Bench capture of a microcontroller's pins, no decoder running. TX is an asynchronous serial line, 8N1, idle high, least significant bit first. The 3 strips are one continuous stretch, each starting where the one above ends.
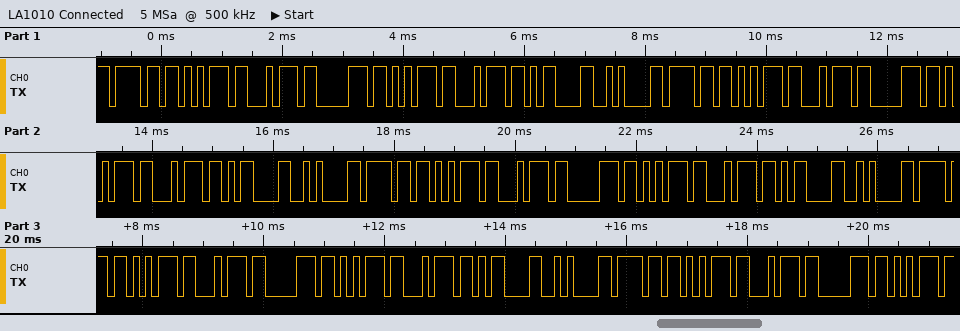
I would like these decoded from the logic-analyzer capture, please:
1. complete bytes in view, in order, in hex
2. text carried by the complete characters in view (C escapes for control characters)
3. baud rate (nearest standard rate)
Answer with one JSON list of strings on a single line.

["6F 75 74 70 75 74 0D 0A 6F 75 74 70 75 74 0D 0A 6F 75 74 70 75 74 0D 0A 6F 75 74 70 75 74 0D 0A 6F 75 74 70 75", "\"output\\r\\noutput\\r\\noutput\\r\\noutput\\r\\noutpu\"", "9600 baud"]
